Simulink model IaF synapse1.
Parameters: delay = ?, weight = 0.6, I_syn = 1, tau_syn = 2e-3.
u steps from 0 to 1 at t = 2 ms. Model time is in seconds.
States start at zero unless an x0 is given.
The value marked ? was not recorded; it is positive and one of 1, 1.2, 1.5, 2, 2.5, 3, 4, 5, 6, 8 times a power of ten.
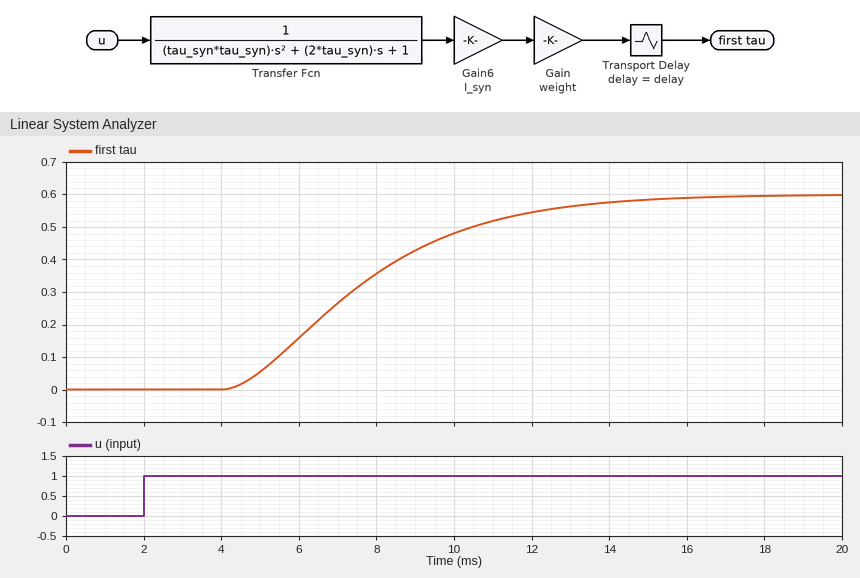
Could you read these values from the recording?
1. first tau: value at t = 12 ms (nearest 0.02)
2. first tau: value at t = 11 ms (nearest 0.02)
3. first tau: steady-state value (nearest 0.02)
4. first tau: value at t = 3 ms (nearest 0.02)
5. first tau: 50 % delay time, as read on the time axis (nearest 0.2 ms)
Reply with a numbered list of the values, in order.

1. 0.54
2. 0.52
3. 0.60
4. 0.00
5. 7.4 ms
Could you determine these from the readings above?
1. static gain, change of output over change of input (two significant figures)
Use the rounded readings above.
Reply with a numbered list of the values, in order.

1. 0.60
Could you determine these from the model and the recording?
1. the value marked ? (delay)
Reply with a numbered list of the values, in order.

1. 0.002
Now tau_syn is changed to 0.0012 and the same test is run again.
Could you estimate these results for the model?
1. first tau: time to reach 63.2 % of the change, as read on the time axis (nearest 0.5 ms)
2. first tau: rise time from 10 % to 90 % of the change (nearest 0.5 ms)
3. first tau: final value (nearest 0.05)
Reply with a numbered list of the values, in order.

1. 6.5 ms
2. 4.0 ms
3. 0.60
